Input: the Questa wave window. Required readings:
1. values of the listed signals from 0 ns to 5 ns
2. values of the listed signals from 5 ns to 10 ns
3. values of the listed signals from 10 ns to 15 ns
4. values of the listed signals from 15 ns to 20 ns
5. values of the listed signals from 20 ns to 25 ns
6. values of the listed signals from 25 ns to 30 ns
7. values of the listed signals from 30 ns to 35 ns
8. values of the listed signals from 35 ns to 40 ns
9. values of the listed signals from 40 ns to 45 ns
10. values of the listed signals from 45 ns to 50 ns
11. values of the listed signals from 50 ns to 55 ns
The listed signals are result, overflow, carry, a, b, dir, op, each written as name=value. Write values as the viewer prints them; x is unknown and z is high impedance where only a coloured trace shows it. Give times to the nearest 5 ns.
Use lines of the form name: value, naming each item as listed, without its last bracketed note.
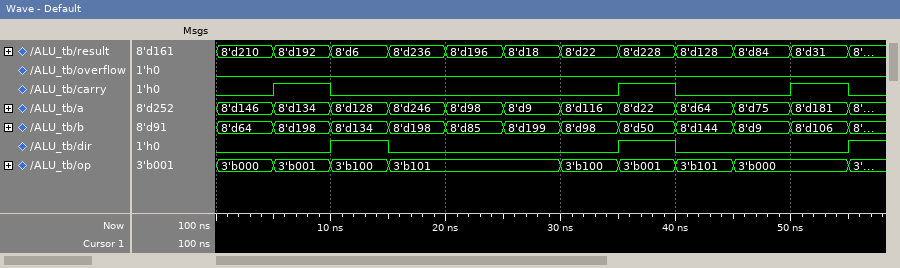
values of the listed signals from 0 ns to 5 ns: result=8'd210, overflow=0, carry=0, a=8'd146, b=8'd64, dir=0, op=3'b000
values of the listed signals from 5 ns to 10 ns: result=8'd192, overflow=0, carry=1, a=8'd134, b=8'd198, dir=0, op=3'b001
values of the listed signals from 10 ns to 15 ns: result=8'd6, overflow=0, carry=0, a=8'd128, b=8'd134, dir=1, op=3'b100
values of the listed signals from 15 ns to 20 ns: result=8'd236, overflow=0, carry=0, a=8'd246, b=8'd198, dir=0, op=3'b101
values of the listed signals from 20 ns to 25 ns: result=8'd196, overflow=0, carry=0, a=8'd98, b=8'd85, dir=0, op=3'b101
values of the listed signals from 25 ns to 30 ns: result=8'd18, overflow=0, carry=0, a=8'd9, b=8'd199, dir=0, op=3'b101
values of the listed signals from 30 ns to 35 ns: result=8'd22, overflow=0, carry=0, a=8'd116, b=8'd98, dir=0, op=3'b100
values of the listed signals from 35 ns to 40 ns: result=8'd228, overflow=0, carry=1, a=8'd22, b=8'd50, dir=1, op=3'b001
values of the listed signals from 40 ns to 45 ns: result=8'd128, overflow=0, carry=0, a=8'd64, b=8'd144, dir=0, op=3'b101
values of the listed signals from 45 ns to 50 ns: result=8'd84, overflow=0, carry=0, a=8'd75, b=8'd9, dir=0, op=3'b000
values of the listed signals from 50 ns to 55 ns: result=8'd31, overflow=0, carry=1, a=8'd181, b=8'd106, dir=0, op=3'b000
